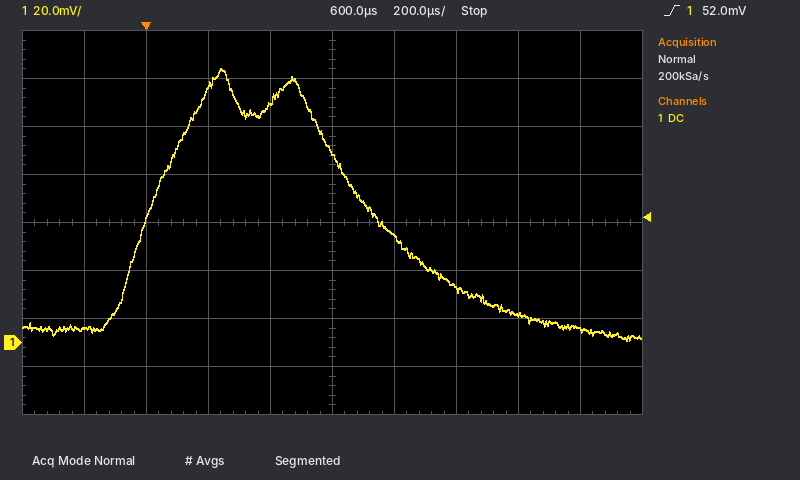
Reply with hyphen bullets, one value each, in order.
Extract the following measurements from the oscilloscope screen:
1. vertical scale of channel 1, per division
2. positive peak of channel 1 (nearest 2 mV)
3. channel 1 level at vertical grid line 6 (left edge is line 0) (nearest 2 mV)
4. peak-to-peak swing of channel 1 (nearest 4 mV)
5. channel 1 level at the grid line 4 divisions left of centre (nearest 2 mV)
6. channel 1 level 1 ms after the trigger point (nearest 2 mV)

- 20 mV
- 114 mV
- 44 mV
- 112 mV
- 6 mV
- 22 mV
